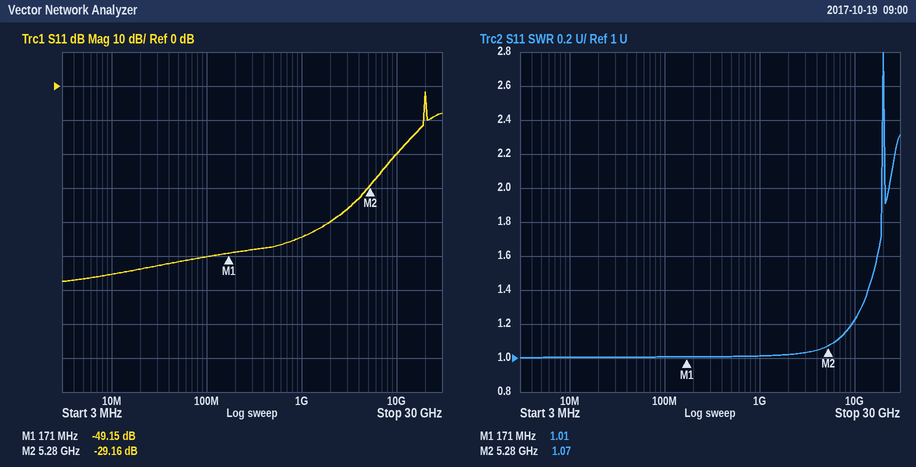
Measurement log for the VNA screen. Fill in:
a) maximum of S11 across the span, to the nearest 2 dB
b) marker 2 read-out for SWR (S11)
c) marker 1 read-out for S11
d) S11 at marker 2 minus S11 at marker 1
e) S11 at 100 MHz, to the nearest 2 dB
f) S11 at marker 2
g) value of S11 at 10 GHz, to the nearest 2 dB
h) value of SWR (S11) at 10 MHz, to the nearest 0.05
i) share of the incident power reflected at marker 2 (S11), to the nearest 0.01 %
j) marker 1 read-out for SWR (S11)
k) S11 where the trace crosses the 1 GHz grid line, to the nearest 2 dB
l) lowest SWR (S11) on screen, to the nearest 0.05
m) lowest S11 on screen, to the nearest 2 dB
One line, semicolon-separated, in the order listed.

-2 dB; 1.07; -49.15 dB; 19.99 dB; -50 dB; -29.16 dB; -20 dB; 1.00; 0.12 %; 1.01; -44 dB; 1.00; -58 dB
